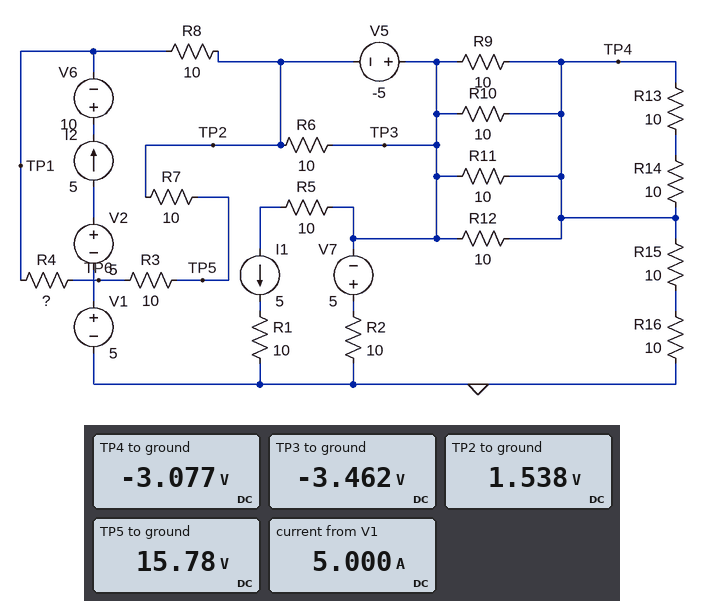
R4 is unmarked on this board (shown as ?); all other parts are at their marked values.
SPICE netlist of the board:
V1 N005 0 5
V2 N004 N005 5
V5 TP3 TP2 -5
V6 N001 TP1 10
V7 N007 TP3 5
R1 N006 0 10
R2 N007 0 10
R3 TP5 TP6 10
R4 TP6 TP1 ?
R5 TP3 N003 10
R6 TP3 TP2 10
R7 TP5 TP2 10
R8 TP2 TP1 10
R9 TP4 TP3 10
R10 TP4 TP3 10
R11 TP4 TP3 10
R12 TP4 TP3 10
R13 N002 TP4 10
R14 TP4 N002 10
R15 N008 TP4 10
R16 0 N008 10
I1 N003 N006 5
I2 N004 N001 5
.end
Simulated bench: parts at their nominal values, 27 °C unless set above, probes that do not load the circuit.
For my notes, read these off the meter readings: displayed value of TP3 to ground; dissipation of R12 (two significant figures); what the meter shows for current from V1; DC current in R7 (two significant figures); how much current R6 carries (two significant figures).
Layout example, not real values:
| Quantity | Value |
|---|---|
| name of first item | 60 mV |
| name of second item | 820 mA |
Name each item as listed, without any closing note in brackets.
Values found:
| Quantity | Value |
|---|---|
| displayed value of TP3 to ground | -3.462 V |
| dissipation of R12 | 15 mW |
| what the meter shows for current from V1 | 5.000 A |
| DC current in R7 | 1.4 A |
| how much current R6 carries | 500 mA |
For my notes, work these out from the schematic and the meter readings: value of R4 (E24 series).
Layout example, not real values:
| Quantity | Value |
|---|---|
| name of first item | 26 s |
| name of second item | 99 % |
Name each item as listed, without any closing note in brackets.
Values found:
| Quantity | Value |
|---|---|
| value of R4 | 5.1 Ω |
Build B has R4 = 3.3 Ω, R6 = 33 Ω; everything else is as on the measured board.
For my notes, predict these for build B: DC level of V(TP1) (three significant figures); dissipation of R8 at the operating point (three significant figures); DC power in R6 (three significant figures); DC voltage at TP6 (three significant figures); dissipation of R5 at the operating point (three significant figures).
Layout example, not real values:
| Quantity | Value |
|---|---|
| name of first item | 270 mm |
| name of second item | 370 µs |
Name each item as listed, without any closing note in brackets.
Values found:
| Quantity | Value |
|---|---|
| DC level of V(TP1) | 36.5 V |
| dissipation of R8 at the operating point | 122 W |
| DC power in R6 | 758 mW |
| DC voltage at TP6 | 31.6 V |
| dissipation of R5 at the operating point | 250 W |
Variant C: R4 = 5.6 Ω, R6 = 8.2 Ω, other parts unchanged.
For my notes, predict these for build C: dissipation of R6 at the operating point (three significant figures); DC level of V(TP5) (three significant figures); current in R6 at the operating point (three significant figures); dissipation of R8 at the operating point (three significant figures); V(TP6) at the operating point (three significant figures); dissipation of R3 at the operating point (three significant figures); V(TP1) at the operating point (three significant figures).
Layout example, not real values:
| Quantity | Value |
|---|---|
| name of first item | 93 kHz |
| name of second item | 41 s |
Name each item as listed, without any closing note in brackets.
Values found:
| Quantity | Value |
|---|---|
| dissipation of R6 at the operating point | 3.05 W |
| DC level of V(TP5) | 15.6 V |
| current in R6 at the operating point | 610 mA |
| dissipation of R8 at the operating point | 129 W |
| V(TP6) at the operating point | 29.6 V |
| dissipation of R3 at the operating point | 19.7 W |
| V(TP1) at the operating point | 37.5 V |
